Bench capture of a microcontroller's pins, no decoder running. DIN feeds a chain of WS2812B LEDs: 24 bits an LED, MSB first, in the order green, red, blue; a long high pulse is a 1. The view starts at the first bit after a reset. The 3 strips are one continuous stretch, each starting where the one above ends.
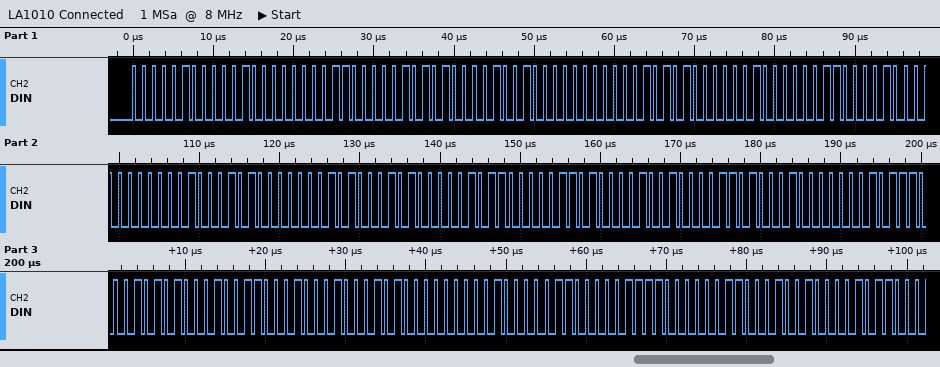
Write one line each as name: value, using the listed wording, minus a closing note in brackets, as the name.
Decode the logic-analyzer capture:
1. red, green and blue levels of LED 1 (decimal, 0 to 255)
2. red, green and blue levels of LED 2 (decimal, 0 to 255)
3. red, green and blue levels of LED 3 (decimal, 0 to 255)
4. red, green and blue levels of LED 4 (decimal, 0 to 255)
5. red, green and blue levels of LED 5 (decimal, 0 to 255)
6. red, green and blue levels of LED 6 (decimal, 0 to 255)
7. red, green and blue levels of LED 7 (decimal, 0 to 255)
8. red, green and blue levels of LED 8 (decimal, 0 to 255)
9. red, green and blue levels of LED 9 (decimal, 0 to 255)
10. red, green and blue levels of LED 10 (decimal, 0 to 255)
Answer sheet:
red, green and blue levels of LED 1: 16, 4, 12
red, green and blue levels of LED 2: 9, 21, 0
red, green and blue levels of LED 3: 2, 21, 6
red, green and blue levels of LED 4: 1, 16, 20
red, green and blue levels of LED 5: 20, 5, 22
red, green and blue levels of LED 6: 9, 13, 13
red, green and blue levels of LED 7: 23, 16, 21
red, green and blue levels of LED 8: 17, 19, 20
red, green and blue levels of LED 9: 6, 1, 15
red, green and blue levels of LED 10: 18, 3, 22
